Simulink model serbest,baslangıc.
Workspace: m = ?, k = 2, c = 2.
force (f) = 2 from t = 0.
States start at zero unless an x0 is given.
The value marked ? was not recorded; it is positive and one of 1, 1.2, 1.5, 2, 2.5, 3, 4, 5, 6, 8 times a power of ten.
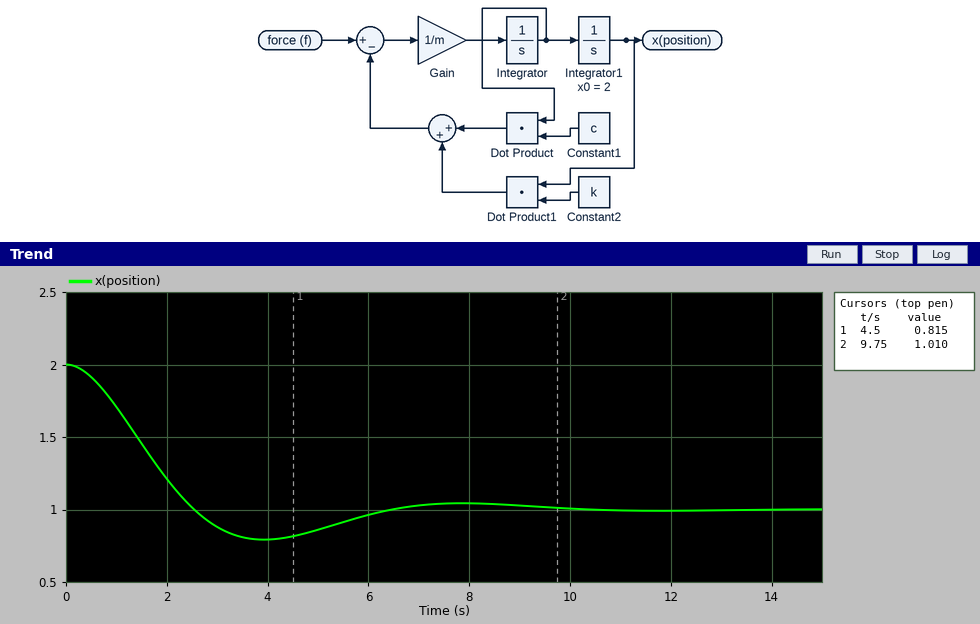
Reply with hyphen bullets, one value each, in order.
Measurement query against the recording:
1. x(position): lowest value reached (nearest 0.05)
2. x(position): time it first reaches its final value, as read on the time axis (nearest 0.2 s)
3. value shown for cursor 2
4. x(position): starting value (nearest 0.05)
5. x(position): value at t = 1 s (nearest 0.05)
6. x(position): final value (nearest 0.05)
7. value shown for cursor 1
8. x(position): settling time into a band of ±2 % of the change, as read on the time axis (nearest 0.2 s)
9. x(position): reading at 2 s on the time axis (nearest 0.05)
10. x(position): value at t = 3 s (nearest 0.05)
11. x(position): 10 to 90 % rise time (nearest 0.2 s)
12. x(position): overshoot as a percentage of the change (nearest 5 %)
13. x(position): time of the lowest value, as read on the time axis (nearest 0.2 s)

- 0.80
- 2.6 s
- 1.010
- 2.00
- 1.70
- 1.00
- 0.815
- 9.4 s
- 1.20
- 0.90
- 1.8 s
- 20 %
- 4.0 s
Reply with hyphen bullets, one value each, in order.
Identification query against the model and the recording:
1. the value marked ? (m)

- 2.5
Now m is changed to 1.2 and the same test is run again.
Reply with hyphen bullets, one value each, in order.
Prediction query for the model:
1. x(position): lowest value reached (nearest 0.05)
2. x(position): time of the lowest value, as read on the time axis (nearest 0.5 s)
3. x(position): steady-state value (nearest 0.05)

- 0.95
- 3.0 s
- 1.00
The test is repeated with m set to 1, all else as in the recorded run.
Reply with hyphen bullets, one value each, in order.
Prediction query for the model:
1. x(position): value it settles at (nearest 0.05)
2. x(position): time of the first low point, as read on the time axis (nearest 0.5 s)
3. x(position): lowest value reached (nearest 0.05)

- 1.00
- 3.0 s
- 0.95
